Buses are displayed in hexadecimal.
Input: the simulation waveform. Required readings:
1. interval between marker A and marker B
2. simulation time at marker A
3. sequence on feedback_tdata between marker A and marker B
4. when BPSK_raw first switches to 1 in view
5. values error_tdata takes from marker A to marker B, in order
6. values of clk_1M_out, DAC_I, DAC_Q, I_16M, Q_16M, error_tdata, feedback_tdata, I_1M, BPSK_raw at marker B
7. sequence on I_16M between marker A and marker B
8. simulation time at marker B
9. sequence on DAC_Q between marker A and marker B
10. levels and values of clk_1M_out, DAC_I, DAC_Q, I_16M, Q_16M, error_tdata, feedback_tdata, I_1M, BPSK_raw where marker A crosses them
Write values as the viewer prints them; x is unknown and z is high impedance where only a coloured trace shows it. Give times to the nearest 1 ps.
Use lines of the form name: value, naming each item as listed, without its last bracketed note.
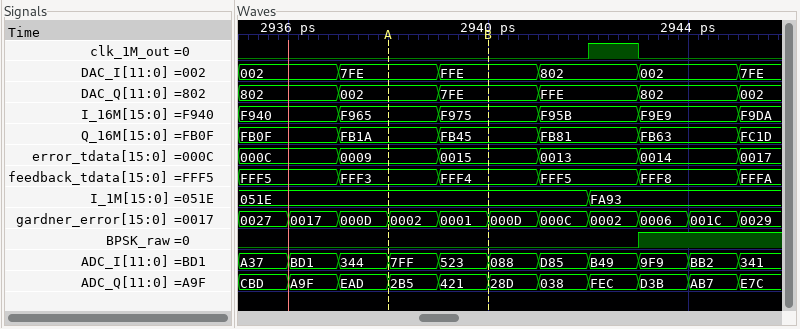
interval between marker A and marker B: 2 ps
simulation time at marker A: 2938 ps
sequence on feedback_tdata between marker A and marker B: FFF3, FFF4
when BPSK_raw first switches to 1 in view: 2943 ps
values error_tdata takes from marker A to marker B, in order: 0009, 0015
values of clk_1M_out, DAC_I, DAC_Q, I_16M, Q_16M, error_tdata, feedback_tdata, I_1M, BPSK_raw at marker B: clk_1M_out=0, DAC_I=FFE, DAC_Q=7FE, I_16M=F975, Q_16M=FB45, error_tdata=0015, feedback_tdata=FFF4, I_1M=051E, BPSK_raw=0
sequence on I_16M between marker A and marker B: F965, F975
simulation time at marker B: 2940 ps
sequence on DAC_Q between marker A and marker B: 002, 7FE
levels and values of clk_1M_out, DAC_I, DAC_Q, I_16M, Q_16M, error_tdata, feedback_tdata, I_1M, BPSK_raw where marker A crosses them: clk_1M_out=0, DAC_I=7FE, DAC_Q=002, I_16M=F965, Q_16M=FB1A, error_tdata=0009, feedback_tdata=FFF3, I_1M=051E, BPSK_raw=0
